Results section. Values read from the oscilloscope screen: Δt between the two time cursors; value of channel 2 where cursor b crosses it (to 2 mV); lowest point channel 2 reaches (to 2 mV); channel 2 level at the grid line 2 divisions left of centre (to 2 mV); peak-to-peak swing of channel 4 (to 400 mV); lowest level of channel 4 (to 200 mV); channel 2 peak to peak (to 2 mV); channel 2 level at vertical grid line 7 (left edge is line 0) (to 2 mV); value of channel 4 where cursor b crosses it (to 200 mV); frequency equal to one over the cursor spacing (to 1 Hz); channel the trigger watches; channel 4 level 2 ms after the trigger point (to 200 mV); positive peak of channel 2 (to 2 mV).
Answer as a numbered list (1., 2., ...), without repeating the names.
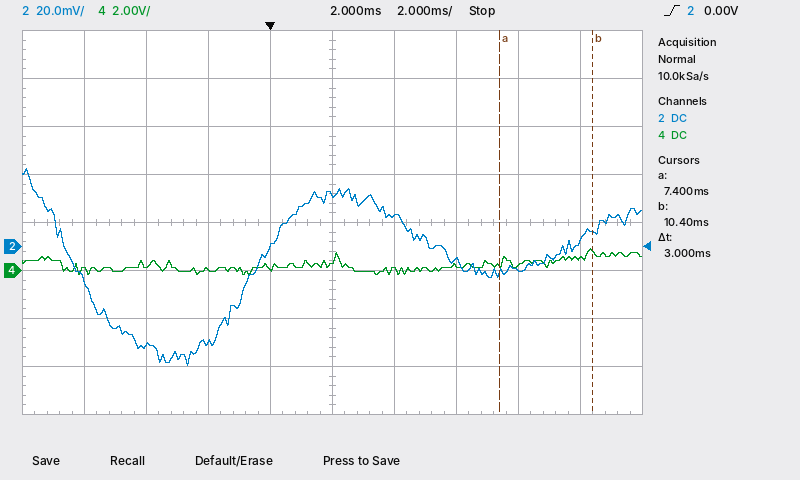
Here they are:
1. 3 ms
2. 6 mV
3. -50 mV
4. -40 mV
5. 1.2 V
6. -200 mV
7. 82 mV
8. -6 mV
9. 800 mV
10. 333 Hz
11. channel 2
12. 400 mV
13. 32 mV
